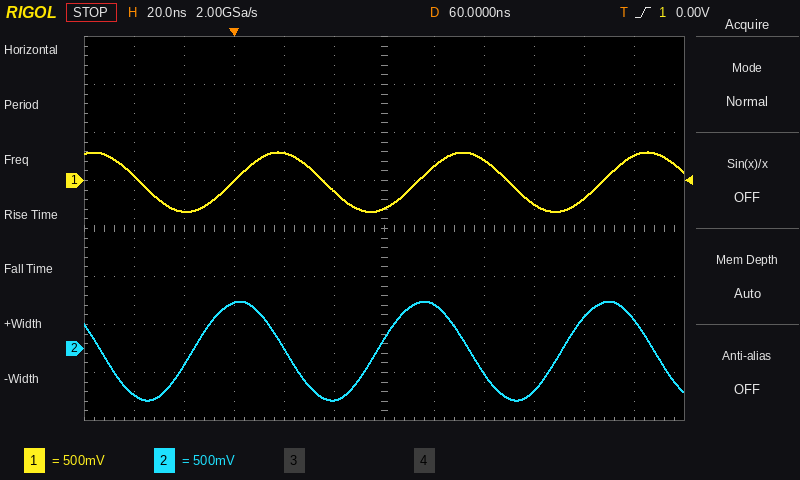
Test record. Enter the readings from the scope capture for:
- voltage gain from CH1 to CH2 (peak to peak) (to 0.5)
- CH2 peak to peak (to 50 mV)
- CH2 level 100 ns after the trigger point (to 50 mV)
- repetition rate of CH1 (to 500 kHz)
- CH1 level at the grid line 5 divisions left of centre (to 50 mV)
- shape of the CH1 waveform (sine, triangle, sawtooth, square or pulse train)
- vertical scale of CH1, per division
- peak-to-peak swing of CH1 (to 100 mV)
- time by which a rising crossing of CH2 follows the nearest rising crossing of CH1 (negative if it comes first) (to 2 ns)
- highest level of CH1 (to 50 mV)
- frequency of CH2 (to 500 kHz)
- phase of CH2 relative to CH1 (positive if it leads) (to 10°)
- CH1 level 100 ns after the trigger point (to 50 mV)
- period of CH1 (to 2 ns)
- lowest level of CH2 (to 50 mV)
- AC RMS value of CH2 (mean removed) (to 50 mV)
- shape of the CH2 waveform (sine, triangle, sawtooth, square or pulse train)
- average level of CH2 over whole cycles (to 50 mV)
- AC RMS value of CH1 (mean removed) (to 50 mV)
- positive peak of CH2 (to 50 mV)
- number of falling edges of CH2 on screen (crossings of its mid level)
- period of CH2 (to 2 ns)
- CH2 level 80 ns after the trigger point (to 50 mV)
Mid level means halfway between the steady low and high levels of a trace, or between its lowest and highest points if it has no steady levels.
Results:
1.5
1.05 V
-250 mV
13.5 MHz
50 mV
sine
500 mV
600 mV
-16 ns
300 mV
13.5 MHz
+80°
200 mV
74 ns
-550 mV
350 mV
sine
0 mV
200 mV
500 mV
4
74 ns
450 mV
